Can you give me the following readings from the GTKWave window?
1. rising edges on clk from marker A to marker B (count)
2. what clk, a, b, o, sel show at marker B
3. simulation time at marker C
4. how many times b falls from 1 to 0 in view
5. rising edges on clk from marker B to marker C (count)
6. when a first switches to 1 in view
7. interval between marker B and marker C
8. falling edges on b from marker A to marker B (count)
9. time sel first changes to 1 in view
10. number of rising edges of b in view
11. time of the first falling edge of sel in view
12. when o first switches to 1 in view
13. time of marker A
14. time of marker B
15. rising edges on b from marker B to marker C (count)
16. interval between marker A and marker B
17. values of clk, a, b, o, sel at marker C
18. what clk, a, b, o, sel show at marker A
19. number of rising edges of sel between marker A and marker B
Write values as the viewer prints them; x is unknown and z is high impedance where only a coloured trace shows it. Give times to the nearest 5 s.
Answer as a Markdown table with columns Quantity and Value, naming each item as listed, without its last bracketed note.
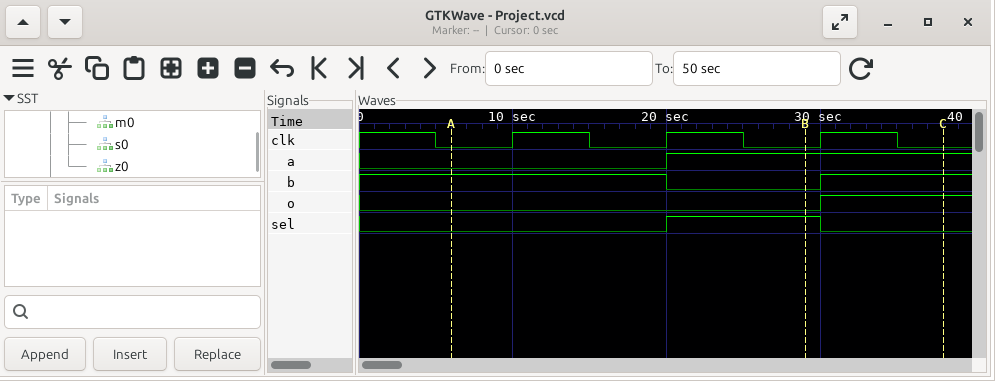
| Quantity | Value |
|---|---|
| rising edges on clk from marker A to marker B | 2 |
| what clk, a, b, o, sel show at marker B | clk=0, a=1, b=0, o=0, sel=1 |
| simulation time at marker C | 40 s |
| how many times b falls from 1 to 0 in view | 1 |
| rising edges on clk from marker B to marker C | 1 |
| when a first switches to 1 in view | 20 s |
| interval between marker B and marker C | 10 s |
| falling edges on b from marker A to marker B | 1 |
| time sel first changes to 1 in view | 20 s |
| number of rising edges of b in view | 1 |
| time of the first falling edge of sel in view | 30 s |
| when o first switches to 1 in view | 30 s |
| time of marker A | 5 s |
| time of marker B | 30 s |
| rising edges on b from marker B to marker C | 1 |
| interval between marker A and marker B | 25 s |
| values of clk, a, b, o, sel at marker C | clk=0, a=1, b=1, o=1, sel=0 |
| what clk, a, b, o, sel show at marker A | clk=0, a=0, b=1, o=0, sel=0 |
| number of rising edges of sel between marker A and marker B | 1 |
